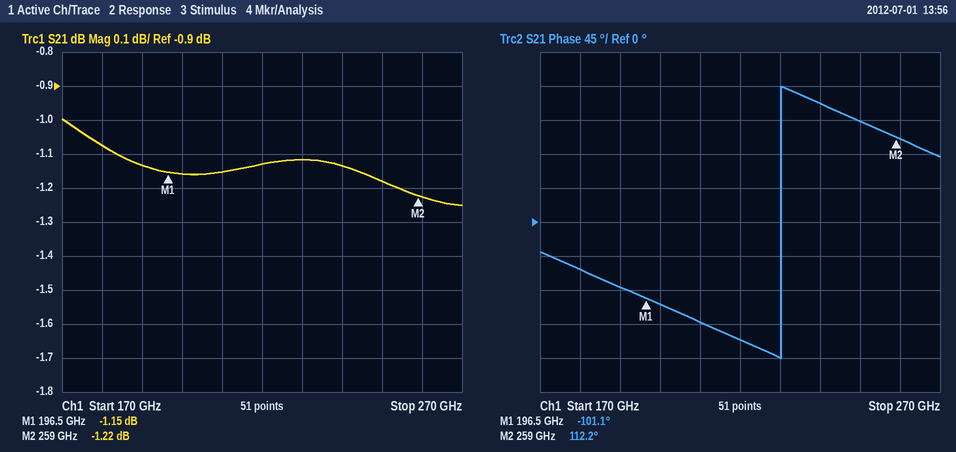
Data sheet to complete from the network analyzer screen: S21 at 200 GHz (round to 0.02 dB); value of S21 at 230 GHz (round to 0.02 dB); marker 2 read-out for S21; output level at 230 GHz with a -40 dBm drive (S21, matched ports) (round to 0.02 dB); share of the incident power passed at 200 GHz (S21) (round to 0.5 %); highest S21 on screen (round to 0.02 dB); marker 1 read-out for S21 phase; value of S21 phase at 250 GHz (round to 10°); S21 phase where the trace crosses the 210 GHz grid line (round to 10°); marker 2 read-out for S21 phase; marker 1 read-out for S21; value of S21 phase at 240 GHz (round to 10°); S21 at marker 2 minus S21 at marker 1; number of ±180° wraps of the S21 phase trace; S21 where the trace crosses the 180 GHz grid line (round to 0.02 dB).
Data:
-1.16 dB
-1.12 dB
-1.22 dB
-41.12 dBm
76.5 %
-1.00 dB
-101.1°
130°
-130°
112.2°
-1.15 dB
160°
-0.07 dB
1
-1.08 dB
